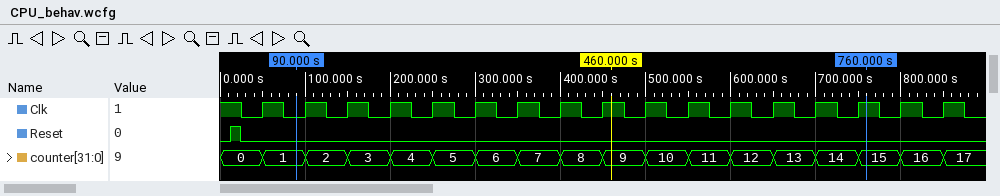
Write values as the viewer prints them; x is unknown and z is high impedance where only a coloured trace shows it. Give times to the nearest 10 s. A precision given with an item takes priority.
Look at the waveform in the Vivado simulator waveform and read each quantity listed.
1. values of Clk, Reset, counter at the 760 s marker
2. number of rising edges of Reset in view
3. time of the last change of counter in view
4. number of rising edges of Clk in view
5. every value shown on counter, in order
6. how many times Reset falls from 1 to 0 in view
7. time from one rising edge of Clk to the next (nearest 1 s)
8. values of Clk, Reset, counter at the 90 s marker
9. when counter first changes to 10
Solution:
Clk=1, Reset=0, counter=15
1
850 s
17
0, 1, 2, 3, 4, 5, 6, 7, 8, 9, 10, 11, 12, 13, 14, 15, 16, 17
1
50 s
Clk=0, Reset=0, counter=1
500 s
